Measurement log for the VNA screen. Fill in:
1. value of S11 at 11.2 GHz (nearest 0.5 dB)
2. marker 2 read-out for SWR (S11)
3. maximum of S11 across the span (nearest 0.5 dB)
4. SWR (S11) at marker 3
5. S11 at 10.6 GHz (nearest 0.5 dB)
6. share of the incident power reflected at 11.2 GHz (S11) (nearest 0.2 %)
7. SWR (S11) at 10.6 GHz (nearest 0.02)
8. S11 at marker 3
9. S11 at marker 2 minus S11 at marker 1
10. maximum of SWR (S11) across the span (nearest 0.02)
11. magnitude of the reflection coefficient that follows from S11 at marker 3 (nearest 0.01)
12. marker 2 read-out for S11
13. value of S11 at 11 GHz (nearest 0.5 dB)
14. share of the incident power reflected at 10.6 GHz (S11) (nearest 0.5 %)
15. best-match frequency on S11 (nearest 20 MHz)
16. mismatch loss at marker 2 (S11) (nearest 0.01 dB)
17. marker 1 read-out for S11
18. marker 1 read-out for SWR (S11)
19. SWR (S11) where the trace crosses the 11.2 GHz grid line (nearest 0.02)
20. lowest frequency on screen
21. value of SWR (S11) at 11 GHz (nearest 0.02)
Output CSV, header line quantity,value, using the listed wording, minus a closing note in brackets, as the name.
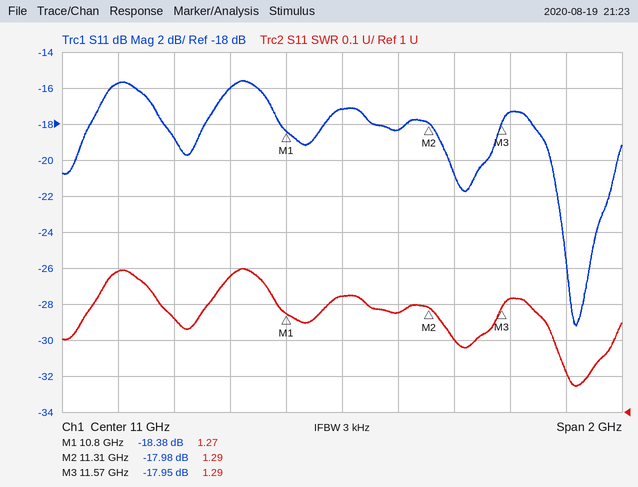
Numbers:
quantity,value
value of S11 at 11.2 GHz,-18.5 dB
marker 2 read-out for SWR,1.29
maximum of S11 across the span,-15.5 dB
SWR (S11) at marker 3,1.29
S11 at 10.6 GHz,-16.0 dB
share of the incident power reflected at 11.2 GHz (S11),1.4 %
SWR (S11) at 10.6 GHz,1.38
S11 at marker 3,-17.95 dB
S11 at marker 2 minus S11 at marker 1,0.40 dB
maximum of SWR (S11) across the span,1.40
magnitude of the reflection coefficient that follows from S11 at marker 3,0.13
marker 2 read-out for S11,-17.98 dB
value of S11 at 11 GHz,-17.0 dB
share of the incident power reflected at 10.6 GHz (S11),2.5 %
best-match frequency on S11,11.84 GHz
mismatch loss at marker 2 (S11),0.07 dB
marker 1 read-out for S11,-18.38 dB
marker 1 read-out for SWR,1.27
SWR (S11) where the trace crosses the 11.2 GHz grid line,1.28
lowest frequency on screen,10 GHz
value of SWR (S11) at 11 GHz,1.32
